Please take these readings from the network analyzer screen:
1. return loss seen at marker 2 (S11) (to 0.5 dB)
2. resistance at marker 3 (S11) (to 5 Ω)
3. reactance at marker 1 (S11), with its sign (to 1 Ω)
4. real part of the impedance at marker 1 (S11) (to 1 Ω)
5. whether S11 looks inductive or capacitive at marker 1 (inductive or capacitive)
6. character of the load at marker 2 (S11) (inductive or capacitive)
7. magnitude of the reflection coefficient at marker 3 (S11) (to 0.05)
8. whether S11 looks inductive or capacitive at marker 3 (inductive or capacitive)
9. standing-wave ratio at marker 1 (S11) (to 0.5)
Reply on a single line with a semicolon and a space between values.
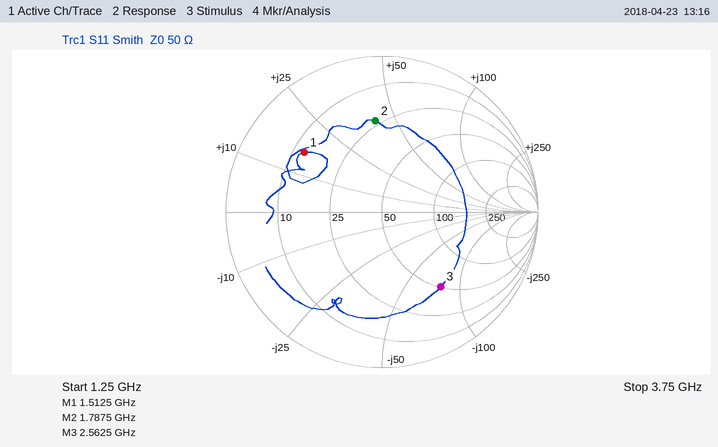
4.5 dB; 50 Ω; +16 Ω; 13 Ω; inductive; inductive; 0.60; capacitive; 4.5
